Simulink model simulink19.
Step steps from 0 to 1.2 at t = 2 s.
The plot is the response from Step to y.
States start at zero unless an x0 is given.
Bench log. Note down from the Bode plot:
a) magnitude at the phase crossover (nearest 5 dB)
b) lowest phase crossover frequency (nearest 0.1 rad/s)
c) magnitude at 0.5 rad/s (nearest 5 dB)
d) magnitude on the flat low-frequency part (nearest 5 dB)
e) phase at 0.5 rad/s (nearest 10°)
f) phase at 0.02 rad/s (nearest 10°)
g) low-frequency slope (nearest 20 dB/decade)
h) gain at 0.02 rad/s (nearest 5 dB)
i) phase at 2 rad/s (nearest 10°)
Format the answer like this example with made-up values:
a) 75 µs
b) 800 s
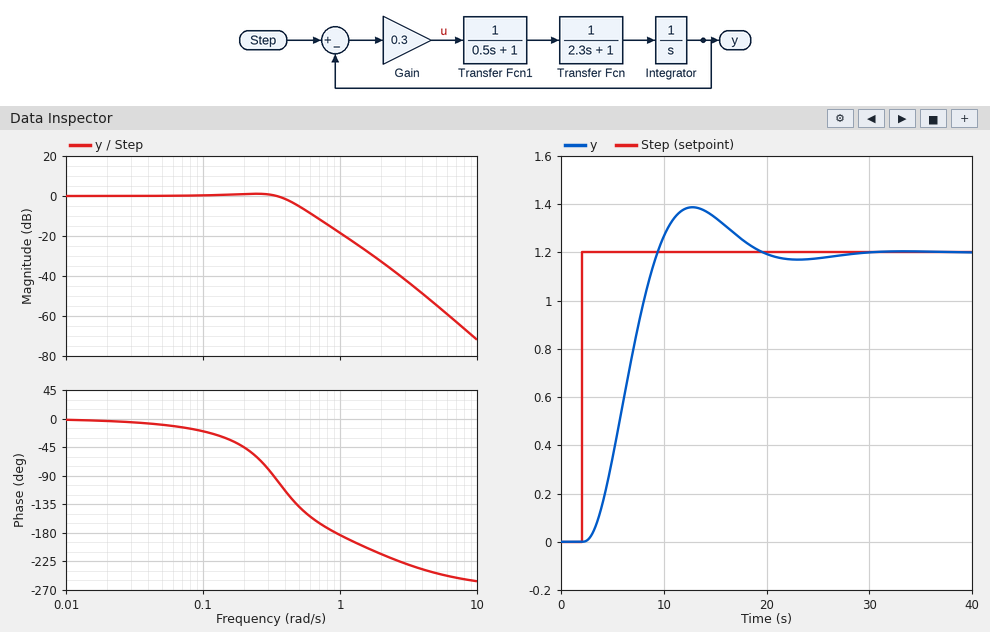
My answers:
a) -15 dB
b) 0.9 rad/s
c) -5 dB
d) 0 dB
e) -140°
f) 0°
g) 0 dB/decade
h) 0 dB
i) -210°
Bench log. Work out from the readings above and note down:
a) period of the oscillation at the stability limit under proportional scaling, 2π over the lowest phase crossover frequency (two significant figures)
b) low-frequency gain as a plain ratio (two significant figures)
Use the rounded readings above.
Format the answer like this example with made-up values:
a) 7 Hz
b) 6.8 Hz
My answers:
a) 7.0 s
b) 1.0
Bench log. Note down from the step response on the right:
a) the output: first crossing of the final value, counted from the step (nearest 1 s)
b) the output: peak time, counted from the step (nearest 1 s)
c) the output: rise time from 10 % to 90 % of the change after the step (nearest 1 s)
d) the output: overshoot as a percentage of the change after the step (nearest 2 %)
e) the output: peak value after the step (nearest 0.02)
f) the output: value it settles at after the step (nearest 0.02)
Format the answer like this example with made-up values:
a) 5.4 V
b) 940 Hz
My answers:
a) 7 s
b) 11 s
c) 5 s
d) 16 %
e) 1.38
f) 1.20
